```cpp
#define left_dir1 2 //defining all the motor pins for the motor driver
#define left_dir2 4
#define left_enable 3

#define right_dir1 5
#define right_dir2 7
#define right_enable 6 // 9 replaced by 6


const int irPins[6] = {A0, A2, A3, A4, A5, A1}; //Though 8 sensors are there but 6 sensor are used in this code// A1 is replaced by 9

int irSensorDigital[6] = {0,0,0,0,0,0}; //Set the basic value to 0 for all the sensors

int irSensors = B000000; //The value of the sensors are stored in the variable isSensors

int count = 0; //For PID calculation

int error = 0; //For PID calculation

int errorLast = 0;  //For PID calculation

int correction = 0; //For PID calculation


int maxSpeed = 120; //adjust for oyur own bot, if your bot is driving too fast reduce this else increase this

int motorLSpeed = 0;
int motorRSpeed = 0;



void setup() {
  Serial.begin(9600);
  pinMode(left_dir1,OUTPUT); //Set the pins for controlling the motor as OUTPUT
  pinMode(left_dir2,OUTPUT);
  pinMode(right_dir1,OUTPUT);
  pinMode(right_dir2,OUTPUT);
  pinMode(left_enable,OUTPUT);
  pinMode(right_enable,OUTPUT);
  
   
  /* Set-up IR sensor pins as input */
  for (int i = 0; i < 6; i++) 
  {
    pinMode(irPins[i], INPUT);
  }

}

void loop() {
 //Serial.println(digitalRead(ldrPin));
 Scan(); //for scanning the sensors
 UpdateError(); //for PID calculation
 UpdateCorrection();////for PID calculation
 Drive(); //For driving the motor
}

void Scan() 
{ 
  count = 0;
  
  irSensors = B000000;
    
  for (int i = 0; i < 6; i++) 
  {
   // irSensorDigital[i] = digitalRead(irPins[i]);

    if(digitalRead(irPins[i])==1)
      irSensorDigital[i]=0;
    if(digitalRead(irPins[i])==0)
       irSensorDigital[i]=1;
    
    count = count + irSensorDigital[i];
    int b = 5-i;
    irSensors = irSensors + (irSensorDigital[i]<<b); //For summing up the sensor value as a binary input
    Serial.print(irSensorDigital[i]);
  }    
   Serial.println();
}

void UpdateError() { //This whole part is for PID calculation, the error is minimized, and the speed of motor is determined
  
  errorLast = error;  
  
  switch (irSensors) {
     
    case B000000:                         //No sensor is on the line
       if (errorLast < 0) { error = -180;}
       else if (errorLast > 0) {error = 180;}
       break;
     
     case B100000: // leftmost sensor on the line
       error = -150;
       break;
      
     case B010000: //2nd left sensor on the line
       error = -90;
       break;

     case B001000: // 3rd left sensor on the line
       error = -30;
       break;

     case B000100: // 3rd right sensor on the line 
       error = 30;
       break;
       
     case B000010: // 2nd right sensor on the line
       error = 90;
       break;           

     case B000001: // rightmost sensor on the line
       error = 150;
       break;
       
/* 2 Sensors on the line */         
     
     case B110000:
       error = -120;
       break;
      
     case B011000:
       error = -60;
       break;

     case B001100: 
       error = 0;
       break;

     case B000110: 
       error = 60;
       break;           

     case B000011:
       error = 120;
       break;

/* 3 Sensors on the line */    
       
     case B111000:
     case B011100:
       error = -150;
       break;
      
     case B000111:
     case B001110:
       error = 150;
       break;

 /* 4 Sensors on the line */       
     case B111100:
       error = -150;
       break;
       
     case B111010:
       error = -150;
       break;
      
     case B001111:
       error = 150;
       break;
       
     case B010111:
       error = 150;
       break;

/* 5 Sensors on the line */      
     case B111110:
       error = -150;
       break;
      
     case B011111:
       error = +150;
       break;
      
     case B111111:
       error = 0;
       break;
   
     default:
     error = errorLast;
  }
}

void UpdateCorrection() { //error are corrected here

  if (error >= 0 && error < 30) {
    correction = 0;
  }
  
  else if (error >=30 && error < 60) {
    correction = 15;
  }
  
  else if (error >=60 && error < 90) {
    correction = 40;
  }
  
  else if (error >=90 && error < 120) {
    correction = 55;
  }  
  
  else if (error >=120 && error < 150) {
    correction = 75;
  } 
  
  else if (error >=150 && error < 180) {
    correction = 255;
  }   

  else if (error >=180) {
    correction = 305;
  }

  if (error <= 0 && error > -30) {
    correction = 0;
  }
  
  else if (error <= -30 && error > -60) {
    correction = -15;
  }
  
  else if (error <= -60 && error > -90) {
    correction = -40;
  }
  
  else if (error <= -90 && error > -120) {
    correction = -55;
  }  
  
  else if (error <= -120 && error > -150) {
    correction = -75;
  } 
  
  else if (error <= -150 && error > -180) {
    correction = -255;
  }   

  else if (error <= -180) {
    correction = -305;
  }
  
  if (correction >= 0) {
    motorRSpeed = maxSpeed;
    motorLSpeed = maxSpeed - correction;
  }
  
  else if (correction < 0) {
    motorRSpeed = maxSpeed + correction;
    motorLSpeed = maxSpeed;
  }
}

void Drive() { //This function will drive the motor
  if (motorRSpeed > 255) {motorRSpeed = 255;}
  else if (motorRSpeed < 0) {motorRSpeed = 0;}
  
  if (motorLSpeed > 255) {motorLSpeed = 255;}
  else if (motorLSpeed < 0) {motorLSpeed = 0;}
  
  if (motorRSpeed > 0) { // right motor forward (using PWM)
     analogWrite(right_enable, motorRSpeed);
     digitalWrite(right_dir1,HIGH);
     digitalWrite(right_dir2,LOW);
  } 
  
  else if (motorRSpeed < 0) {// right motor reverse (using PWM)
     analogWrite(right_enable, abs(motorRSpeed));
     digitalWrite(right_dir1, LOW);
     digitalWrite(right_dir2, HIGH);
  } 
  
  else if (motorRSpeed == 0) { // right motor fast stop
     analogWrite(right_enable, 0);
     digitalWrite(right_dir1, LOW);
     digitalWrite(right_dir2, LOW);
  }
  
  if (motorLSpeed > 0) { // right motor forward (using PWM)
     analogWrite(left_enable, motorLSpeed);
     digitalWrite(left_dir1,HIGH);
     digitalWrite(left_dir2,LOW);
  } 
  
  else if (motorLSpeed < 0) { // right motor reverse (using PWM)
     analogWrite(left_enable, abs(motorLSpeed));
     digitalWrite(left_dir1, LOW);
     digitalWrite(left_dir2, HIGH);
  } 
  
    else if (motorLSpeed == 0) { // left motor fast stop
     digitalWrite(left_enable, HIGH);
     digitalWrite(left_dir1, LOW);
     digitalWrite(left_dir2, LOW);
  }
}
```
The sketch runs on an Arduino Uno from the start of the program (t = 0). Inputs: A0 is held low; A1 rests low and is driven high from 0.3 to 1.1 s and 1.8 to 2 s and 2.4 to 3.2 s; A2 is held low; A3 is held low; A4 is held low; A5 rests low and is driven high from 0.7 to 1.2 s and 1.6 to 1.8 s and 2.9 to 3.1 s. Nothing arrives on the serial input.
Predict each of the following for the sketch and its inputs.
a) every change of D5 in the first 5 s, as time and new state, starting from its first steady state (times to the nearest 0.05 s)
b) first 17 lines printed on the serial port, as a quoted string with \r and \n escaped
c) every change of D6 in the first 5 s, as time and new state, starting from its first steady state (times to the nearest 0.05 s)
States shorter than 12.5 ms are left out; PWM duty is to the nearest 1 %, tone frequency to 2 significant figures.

0 s high; 0.3 s low; 1.2 s high; 1.8 s low; 2 s high; 2.4 s low; 3.2 s high
"111111\r\n111111\r\n111111\r\n111111\r\n111111\r\n111111\r\n111111\r\n111111\r\n111111\r\n111111\r\n111111\r\n111111\r\n111111\r\n111111\r\n111111\r\n111111\r\n111111\r\n"
0 s PWM 47 %; 0.3 s low; 1.2 s PWM 47 %; 1.8 s low; 2 s PWM 47 %; 2.4 s low; 3.2 s PWM 47 %
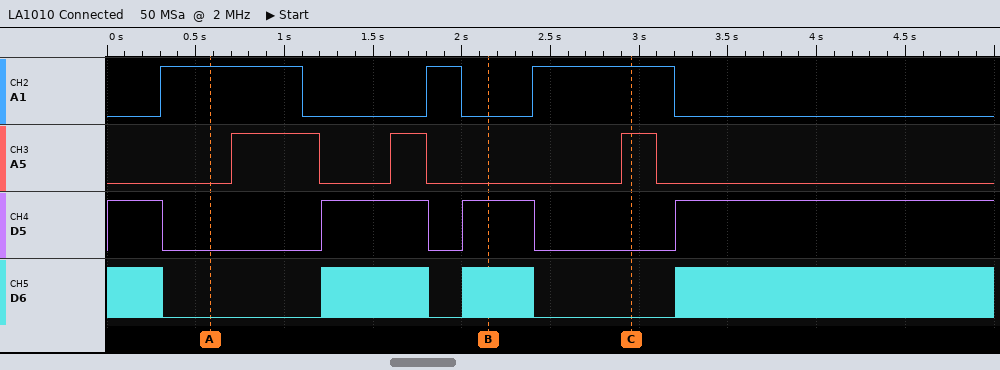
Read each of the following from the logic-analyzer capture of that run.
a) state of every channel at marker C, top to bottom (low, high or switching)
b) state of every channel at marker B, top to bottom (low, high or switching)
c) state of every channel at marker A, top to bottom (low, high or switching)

A1 high, A5 high, D5 low, D6 low
A1 low, A5 low, D5 high, D6 switching
A1 high, A5 low, D5 low, D6 low
